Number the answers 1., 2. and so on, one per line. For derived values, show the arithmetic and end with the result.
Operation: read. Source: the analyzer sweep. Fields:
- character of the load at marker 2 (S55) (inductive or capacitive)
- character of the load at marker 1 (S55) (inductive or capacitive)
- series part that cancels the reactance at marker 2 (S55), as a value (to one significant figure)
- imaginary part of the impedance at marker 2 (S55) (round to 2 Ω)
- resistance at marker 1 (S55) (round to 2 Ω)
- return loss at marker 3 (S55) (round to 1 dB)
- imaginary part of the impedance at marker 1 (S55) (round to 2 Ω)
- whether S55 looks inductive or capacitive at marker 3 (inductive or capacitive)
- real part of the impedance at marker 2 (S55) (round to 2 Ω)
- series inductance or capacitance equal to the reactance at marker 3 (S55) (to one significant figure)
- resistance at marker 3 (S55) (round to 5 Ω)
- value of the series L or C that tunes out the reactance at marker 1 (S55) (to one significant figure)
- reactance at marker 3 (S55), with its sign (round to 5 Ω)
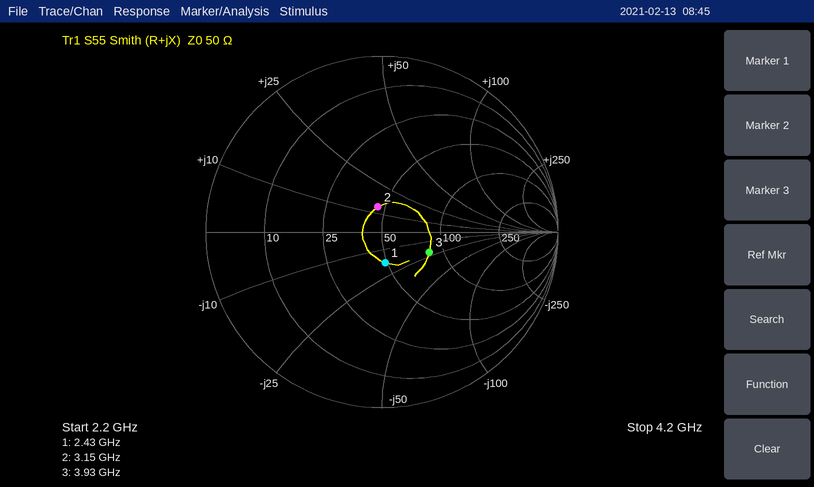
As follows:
1. inductive
2. capacitive
3. C = 1/(2π × 3.15 GHz × 14 Ω) ≈ 4 pF
4. +14 Ω
5. 48 Ω
6. 11 dB
7. -18 Ω
8. capacitive
9. 46 Ω
10. C = 1/(2π × 3.93 GHz × 20 Ω) ≈ 2 pF
11. 85 Ω
12. L = 18 Ω/(2π × 2.43 GHz) ≈ 1 nH
13. -20 Ω
